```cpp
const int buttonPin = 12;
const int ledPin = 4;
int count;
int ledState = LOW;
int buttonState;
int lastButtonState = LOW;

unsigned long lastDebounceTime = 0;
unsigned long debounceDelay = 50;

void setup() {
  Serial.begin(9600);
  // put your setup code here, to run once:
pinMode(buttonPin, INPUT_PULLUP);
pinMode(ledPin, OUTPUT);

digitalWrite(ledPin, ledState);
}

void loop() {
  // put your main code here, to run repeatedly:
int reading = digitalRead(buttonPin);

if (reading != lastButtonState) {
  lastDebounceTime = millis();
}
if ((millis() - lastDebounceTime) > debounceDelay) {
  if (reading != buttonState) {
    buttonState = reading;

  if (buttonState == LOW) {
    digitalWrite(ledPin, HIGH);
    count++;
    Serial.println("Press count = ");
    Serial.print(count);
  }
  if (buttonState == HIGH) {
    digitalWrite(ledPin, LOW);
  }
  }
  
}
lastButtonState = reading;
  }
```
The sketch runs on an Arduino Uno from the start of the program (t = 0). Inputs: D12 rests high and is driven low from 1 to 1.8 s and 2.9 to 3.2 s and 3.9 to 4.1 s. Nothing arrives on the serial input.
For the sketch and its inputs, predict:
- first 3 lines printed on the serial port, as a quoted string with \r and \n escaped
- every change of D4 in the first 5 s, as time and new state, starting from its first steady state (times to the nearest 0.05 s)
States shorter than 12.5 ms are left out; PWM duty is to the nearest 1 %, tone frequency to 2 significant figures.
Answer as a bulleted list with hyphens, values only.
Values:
- "Press count = \r\n1Press count = \r\n2Press count = \r\n"
- 0 s low; 1.05 s high; 1.85 s low; 2.95 s high; 3.25 s low; 3.95 s high; 4.15 s low
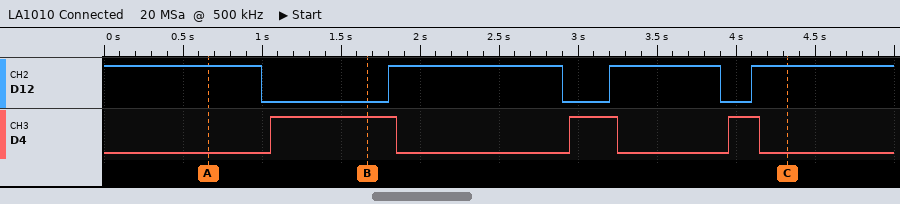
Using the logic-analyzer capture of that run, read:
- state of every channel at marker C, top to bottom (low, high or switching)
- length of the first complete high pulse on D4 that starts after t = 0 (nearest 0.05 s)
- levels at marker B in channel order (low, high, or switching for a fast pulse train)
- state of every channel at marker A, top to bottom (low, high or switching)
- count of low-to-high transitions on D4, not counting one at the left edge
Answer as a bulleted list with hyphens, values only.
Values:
- D12 high, D4 low
- 0.80 s
- D12 low, D4 high
- D12 high, D4 low
- 3
